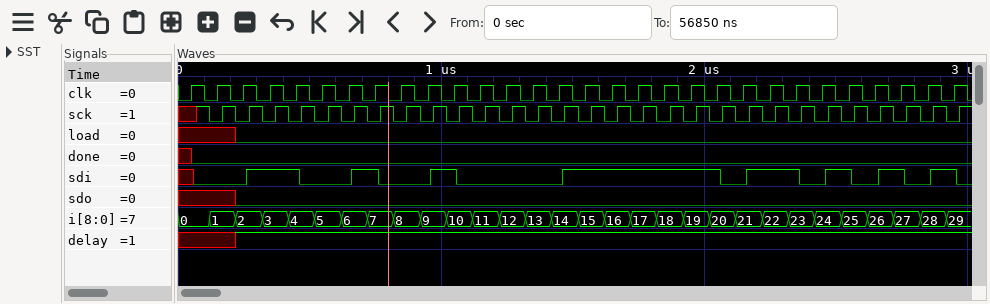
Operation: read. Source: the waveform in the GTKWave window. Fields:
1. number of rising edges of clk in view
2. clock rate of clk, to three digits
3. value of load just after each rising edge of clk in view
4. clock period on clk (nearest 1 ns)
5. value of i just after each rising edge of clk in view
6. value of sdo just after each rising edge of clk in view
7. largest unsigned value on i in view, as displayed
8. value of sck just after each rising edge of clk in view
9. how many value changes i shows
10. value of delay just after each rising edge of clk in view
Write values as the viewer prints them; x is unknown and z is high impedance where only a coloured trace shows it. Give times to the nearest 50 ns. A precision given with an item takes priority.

30
10.0 MHz
x x 0 0 0 0 0 0 0 0 0 0 0 0 0 0 0 0 0 0 0 0 0 0 0 0 0 0 0 0
100 ns
0, 1, 2, 3, 4, 5, 6, 7, 8, 9, 10, 11, 12, 13, 14, 15, 16, 17, 18, 19, 20, 21, 22, 23, 24, 25, 26, 27, 28, 29
x x 0 0 0 0 0 0 0 0 0 0 0 0 0 0 0 0 0 0 0 0 0 0 0 0 0 0 0 0
29
x 0 0 0 0 0 0 0 0 0 0 0 0 0 0 0 0 0 0 0 0 0 0 0 0 0 0 0 0 0
29
x x 1 1 1 1 1 1 1 1 1 1 1 1 1 1 1 1 1 1 1 1 1 1 1 1 1 1 1 1
